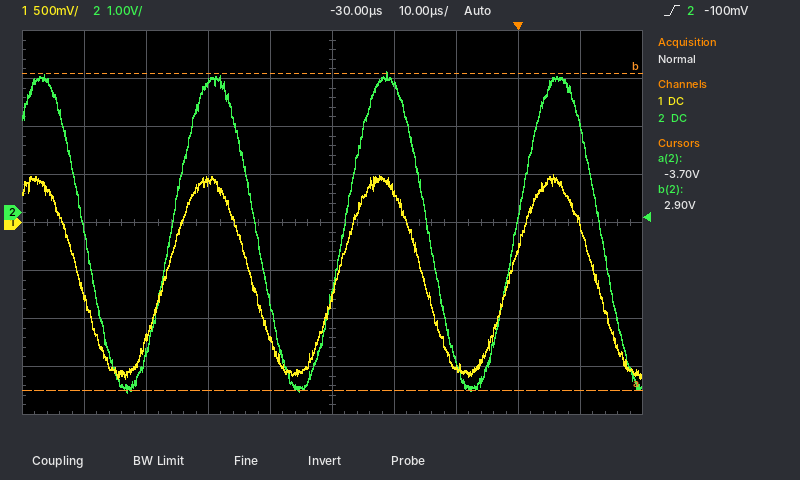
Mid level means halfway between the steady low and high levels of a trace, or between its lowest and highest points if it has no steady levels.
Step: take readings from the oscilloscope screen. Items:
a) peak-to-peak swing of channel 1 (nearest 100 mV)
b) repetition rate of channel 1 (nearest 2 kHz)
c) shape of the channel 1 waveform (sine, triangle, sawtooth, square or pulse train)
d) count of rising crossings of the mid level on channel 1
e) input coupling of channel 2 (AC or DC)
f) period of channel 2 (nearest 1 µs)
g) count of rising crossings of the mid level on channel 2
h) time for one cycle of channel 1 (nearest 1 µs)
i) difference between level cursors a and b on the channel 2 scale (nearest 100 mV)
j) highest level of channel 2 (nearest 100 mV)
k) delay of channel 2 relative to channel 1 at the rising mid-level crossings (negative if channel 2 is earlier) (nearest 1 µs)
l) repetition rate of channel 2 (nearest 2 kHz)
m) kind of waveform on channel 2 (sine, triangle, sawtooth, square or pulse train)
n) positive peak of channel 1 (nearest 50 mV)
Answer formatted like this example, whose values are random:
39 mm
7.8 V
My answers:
2.10 V
36 kHz
sine
3
DC
28 µs
3
28 µs
6.6 V
2.9 V
+1 µs
36 kHz
sine
500 mV
